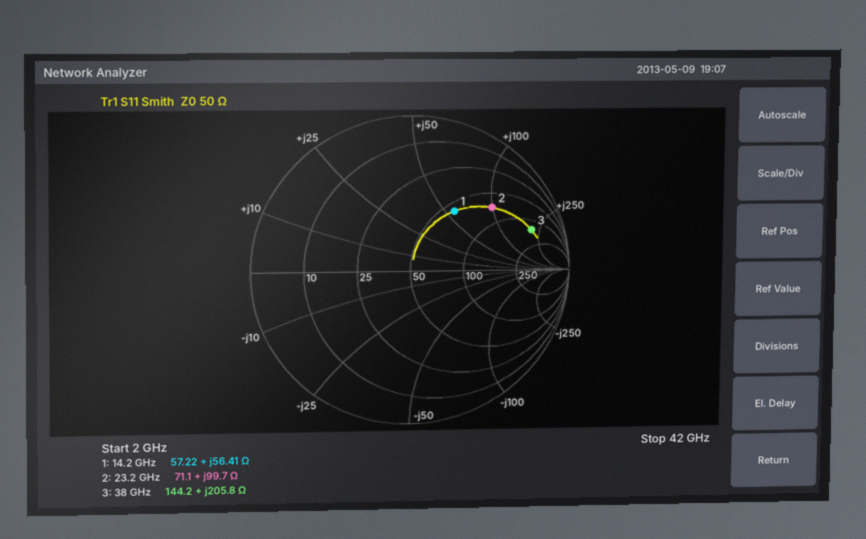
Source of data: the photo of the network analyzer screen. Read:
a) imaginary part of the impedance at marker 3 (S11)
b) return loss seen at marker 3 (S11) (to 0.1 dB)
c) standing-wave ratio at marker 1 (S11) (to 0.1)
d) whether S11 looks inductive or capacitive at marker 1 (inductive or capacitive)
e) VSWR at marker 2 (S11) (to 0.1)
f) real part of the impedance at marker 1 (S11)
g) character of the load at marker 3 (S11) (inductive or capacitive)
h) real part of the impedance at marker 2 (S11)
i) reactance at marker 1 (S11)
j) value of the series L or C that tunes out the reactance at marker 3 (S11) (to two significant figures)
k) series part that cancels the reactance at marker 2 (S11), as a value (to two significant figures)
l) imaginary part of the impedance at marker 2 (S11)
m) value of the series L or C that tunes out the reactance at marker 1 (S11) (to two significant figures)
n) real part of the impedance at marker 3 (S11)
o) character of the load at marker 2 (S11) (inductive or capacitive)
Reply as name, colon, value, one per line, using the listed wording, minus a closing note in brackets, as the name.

imaginary part of the impedance at marker 3: +205.8 Ω
return loss seen at marker 3 (S11): 1.9 dB
standing-wave ratio at marker 1 (S11): 2.8
whether S11 looks inductive or capacitive at marker 1: inductive
VSWR at marker 2 (S11): 4.7
real part of the impedance at marker 1: 57.22 Ω
character of the load at marker 3 (S11): inductive
real part of the impedance at marker 2: 71.1 Ω
reactance at marker 1: +56.41 Ω
value of the series L or C that tunes out the reactance at marker 3 (S11): 20 fF
series part that cancels the reactance at marker 2 (S11), as a value: 69 fF
imaginary part of the impedance at marker 2: +99.7 Ω
value of the series L or C that tunes out the reactance at marker 1 (S11): 200 fF
real part of the impedance at marker 3: 144.2 Ω
character of the load at marker 2 (S11): inductive
